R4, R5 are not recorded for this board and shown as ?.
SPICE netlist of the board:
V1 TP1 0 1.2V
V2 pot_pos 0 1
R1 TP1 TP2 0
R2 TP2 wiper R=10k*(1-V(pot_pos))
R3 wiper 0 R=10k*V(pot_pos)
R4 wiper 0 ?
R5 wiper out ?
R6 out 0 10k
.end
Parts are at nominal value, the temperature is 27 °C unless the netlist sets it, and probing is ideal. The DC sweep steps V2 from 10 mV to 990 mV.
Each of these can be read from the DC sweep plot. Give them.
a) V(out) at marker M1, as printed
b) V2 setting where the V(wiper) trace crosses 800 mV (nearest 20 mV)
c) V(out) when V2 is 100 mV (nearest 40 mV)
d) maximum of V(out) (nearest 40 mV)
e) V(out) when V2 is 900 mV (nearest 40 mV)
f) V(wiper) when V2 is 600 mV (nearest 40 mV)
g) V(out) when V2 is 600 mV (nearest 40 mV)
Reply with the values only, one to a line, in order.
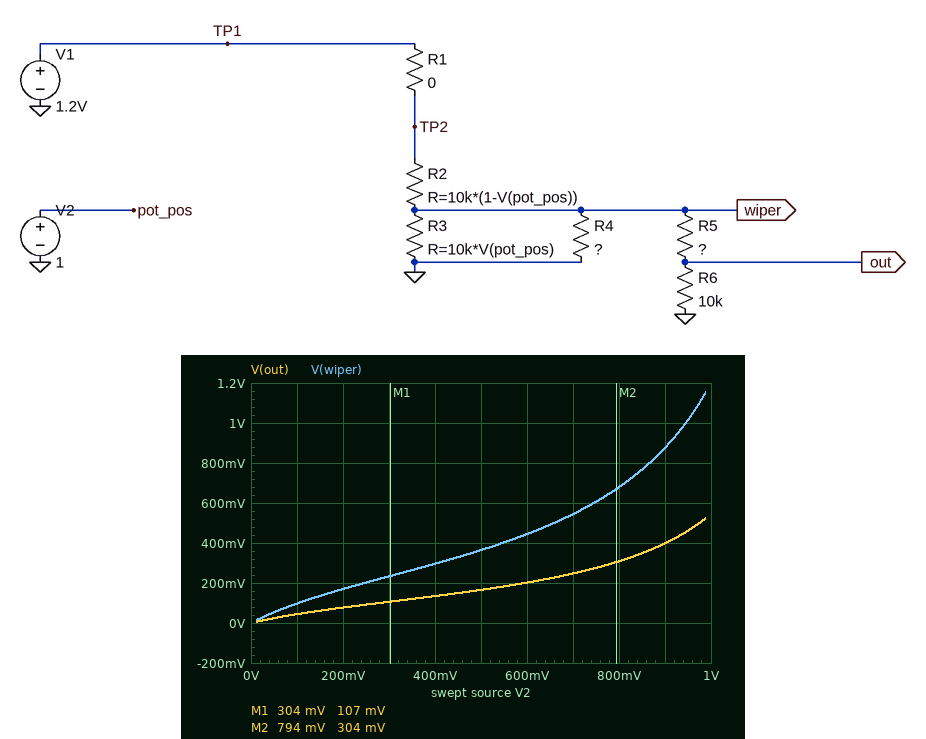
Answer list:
107 mV
860 mV
40 mV
520 mV
400 mV
440 mV
200 mV
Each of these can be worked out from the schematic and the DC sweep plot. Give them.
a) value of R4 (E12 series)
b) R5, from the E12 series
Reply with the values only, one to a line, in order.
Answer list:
4.7 kΩ
12 kΩ
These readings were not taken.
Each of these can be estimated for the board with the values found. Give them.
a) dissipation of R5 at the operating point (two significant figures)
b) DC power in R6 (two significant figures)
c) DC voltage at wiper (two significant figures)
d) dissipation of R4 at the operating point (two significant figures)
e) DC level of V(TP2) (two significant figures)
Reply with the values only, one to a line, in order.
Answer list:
36 µW
30 µW
1.2 V
310 µW
1.2 V
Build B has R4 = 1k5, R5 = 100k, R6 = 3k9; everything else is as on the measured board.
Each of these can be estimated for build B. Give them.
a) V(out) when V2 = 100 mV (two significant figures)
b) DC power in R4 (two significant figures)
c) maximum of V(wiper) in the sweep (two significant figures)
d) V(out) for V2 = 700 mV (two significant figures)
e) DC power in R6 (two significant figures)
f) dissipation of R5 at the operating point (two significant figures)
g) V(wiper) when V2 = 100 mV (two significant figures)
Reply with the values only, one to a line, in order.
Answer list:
2.8 mV
960 µW
1.1 V
13 mV
520 nW
13 µW
75 mV
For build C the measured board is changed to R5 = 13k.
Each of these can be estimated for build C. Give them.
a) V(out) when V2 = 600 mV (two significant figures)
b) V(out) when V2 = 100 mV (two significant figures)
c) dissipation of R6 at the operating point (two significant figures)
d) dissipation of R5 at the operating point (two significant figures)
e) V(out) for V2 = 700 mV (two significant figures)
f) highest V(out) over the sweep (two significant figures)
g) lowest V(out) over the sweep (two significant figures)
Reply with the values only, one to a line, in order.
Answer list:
190 mV
42 mV
27 µW
35 µW
240 mV
500 mV
5.1 mV
